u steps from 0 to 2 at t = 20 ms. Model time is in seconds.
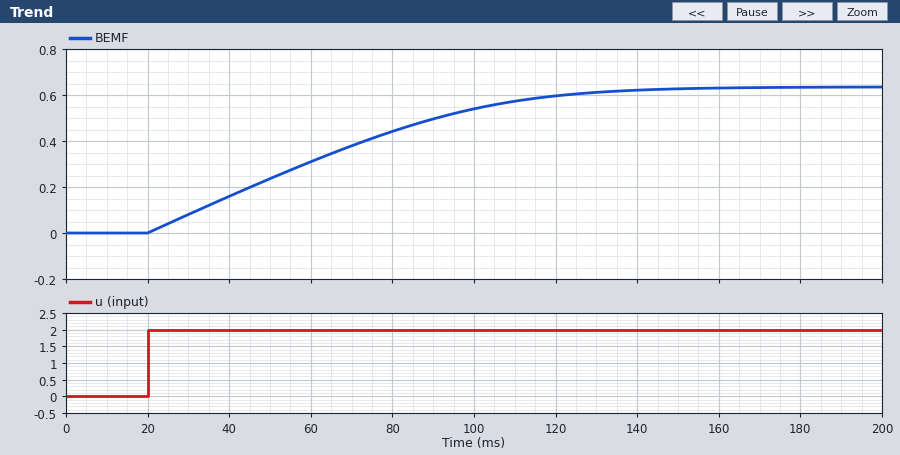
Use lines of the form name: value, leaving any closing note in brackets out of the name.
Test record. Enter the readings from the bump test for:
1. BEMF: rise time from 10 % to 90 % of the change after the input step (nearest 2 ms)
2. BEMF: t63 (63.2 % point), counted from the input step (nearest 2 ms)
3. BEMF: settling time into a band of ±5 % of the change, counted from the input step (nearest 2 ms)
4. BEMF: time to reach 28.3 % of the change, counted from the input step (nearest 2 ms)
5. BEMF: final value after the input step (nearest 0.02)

BEMF: rise time from 10 % to 90 % of the change after the input step: 82 ms
BEMF: t63 (63.2 % point), counted from the input step: 54 ms
BEMF: settling time into a band of ±5 % of the change, counted from the input step: 104 ms
BEMF: time to reach 28.3 % of the change, counted from the input step: 22 ms
BEMF: final value after the input step: 0.64
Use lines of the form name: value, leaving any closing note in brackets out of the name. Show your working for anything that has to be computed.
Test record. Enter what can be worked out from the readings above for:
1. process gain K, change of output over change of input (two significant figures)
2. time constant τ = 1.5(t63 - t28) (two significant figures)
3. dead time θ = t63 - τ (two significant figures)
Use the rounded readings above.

process gain K, change of output over change of input: (0.64 - 0) / 2 = 0.32
time constant τ = 1.5(t63 - t28): 1.5 × (54 - 22) = 48 ms
dead time θ = t63 - τ: 54 - 48 = 6.0 ms
